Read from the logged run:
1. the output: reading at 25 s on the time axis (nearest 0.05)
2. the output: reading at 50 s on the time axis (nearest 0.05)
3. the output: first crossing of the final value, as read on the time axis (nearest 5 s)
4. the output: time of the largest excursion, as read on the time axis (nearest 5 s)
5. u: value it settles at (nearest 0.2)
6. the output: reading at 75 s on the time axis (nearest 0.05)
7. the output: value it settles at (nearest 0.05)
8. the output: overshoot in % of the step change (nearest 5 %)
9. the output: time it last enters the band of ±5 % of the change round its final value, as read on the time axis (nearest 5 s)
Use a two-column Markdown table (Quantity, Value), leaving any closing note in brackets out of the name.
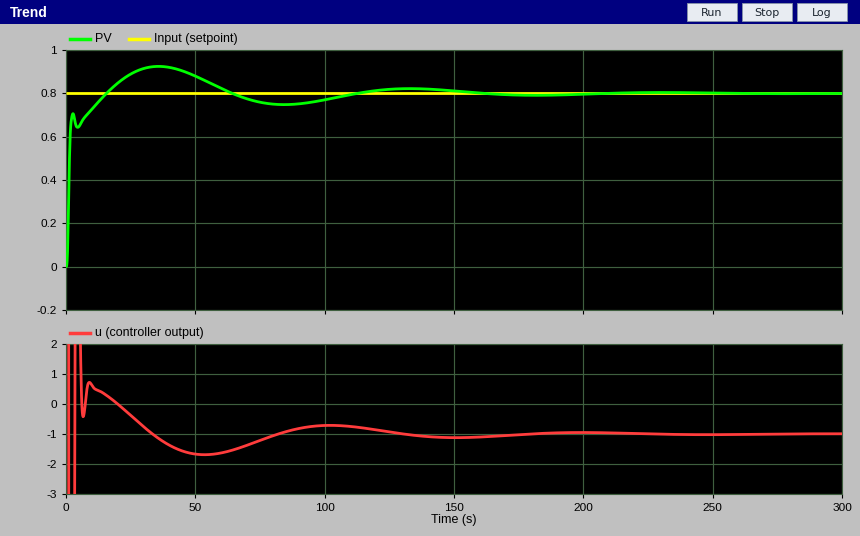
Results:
| Quantity | Value |
|---|---|
| the output: reading at 25 s on the time axis | 0.90 |
| the output: reading at 50 s on the time axis | 0.90 |
| the output: first crossing of the final value, as read on the time axis | 15 s |
| the output: time of the largest excursion, as read on the time axis | 35 s |
| u: value it settles at | -1.0 |
| the output: reading at 75 s on the time axis | 0.75 |
| the output: value it settles at | 0.80 |
| the output: overshoot in % of the step change | 15 % |
| the output: time it last enters the band of ±5 % of the change round its final value, as read on the time axis | 95 s |
